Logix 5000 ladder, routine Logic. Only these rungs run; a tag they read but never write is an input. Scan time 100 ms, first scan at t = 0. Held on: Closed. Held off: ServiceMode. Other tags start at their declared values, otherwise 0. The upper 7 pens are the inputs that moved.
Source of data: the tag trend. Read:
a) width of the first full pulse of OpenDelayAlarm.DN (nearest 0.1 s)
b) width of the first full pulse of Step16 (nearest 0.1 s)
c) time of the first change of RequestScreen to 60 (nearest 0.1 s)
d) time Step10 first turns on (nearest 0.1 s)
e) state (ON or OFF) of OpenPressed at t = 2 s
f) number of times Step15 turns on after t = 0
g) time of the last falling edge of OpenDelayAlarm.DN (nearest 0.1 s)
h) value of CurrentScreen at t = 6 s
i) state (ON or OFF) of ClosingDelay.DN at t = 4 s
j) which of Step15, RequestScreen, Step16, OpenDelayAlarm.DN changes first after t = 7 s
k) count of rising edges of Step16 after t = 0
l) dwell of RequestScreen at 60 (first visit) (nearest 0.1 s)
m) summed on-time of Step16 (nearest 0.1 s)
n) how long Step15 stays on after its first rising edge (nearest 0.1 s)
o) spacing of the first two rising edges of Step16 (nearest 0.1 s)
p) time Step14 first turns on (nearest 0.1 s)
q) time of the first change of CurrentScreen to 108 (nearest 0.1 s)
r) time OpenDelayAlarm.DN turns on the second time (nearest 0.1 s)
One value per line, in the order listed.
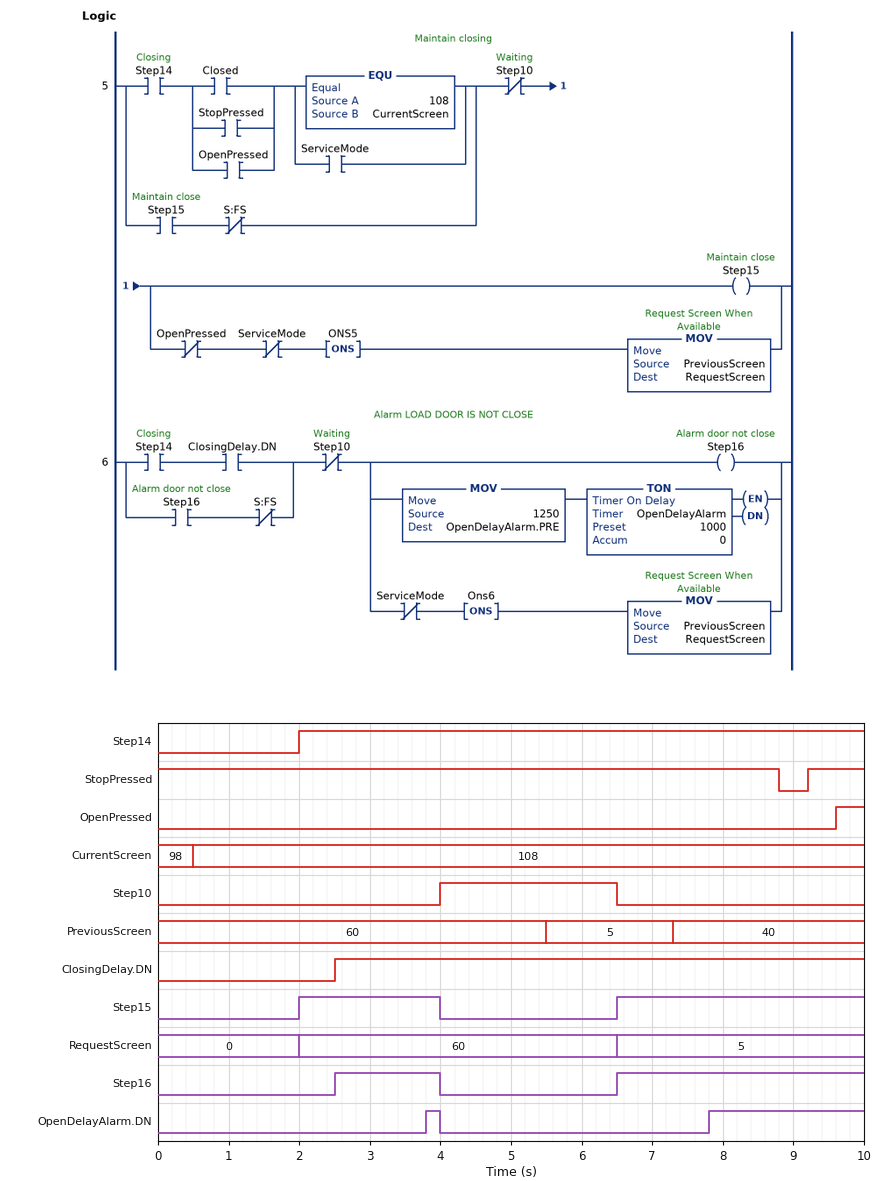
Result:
0.2 s
1.5 s
2.0 s
4.0 s
OFF
2
4.0 s
108
ON
OpenDelayAlarm.DN
2
4.5 s
5.0 s
2.0 s
4.0 s
2.0 s
0.5 s
7.8 s
